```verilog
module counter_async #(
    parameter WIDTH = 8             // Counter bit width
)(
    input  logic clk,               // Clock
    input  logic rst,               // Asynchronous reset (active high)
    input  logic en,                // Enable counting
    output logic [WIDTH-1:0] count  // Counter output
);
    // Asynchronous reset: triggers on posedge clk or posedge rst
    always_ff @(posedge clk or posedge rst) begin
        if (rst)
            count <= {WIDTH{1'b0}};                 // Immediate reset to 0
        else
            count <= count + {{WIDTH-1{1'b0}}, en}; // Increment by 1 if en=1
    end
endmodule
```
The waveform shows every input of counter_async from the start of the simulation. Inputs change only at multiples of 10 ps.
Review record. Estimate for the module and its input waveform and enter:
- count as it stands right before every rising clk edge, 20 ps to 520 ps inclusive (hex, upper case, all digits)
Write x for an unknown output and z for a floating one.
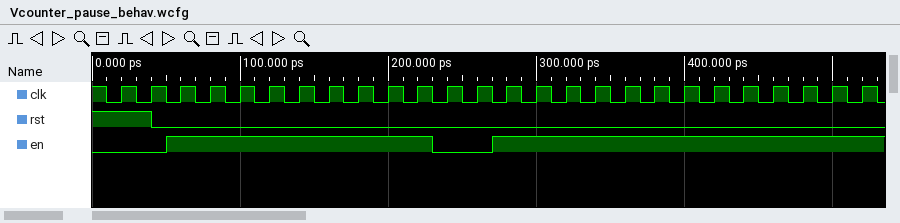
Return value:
00, 00, 00, 01, 02, 03, 04, 05, 06, 07, 08, 09, 09, 09, 0A, 0B, 0C, 0D, 0E, 0F, 10, 11, 12, 13, 14, 15
